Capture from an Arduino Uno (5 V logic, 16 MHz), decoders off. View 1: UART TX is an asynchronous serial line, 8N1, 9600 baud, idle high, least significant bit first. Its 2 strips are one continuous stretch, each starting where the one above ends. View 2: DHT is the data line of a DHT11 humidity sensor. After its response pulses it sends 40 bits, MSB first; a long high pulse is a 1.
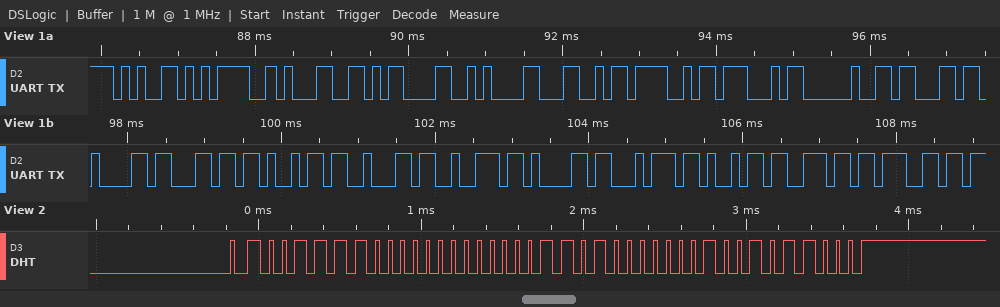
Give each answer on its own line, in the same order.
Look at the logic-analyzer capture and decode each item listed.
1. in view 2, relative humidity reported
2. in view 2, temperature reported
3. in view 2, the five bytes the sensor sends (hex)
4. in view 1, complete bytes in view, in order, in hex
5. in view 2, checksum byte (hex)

60 %
26.2 °C
3C 00 1A 02 58
65 3D 31 0D 0A 4C 4F 47 20 63 61 6C 69 62 72 61 74 69 6E 67
0x58
